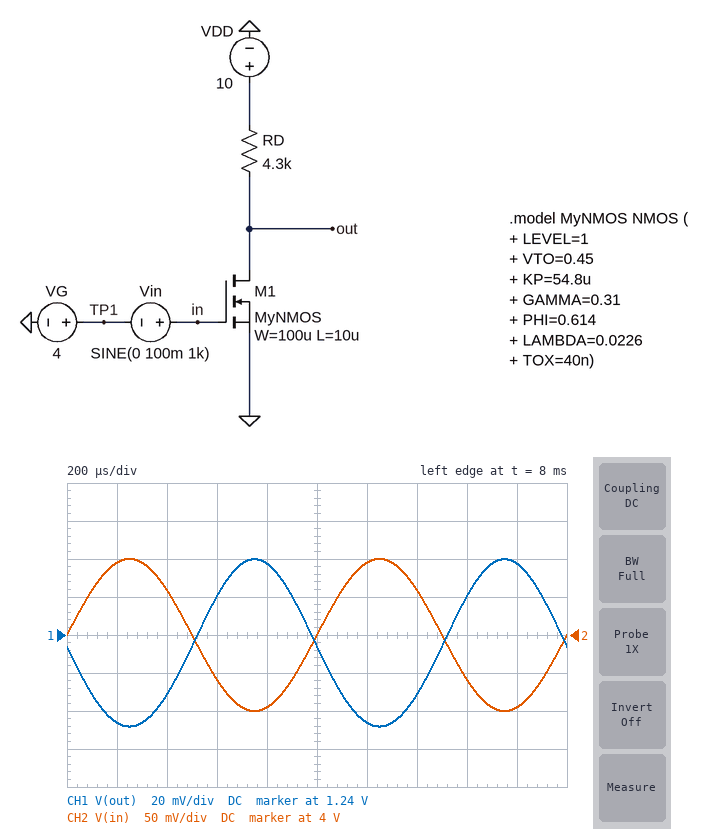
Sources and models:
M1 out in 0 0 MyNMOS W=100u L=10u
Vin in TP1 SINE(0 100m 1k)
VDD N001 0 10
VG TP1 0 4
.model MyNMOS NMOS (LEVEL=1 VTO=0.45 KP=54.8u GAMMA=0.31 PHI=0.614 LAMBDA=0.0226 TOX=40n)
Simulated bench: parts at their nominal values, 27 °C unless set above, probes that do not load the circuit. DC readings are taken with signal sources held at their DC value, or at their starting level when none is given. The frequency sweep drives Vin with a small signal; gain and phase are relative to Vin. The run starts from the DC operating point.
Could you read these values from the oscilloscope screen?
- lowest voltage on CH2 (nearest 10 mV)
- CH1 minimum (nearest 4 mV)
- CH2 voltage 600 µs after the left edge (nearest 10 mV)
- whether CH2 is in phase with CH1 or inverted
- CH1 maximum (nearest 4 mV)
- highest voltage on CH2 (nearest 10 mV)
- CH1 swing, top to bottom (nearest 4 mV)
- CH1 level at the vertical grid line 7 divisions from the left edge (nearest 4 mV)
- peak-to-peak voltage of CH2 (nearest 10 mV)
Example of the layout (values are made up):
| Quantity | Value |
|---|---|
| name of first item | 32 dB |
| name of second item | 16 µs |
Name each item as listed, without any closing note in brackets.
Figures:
| Quantity | Value |
|---|---|
| lowest voltage on CH2 | 3.90 V |
| CH1 minimum | 1.192 V |
| CH2 voltage 600 µs after the left edge | 3.94 V |
| whether CH2 is in phase with CH1 or inverted | inverted |
| CH1 maximum | 1.280 V |
| highest voltage on CH2 | 4.10 V |
| CH1 swing, top to bottom | 88 mV |
| CH1 level at the vertical grid line 7 divisions from the left edge | 1.208 V |
| peak-to-peak voltage of CH2 | 200 mV |
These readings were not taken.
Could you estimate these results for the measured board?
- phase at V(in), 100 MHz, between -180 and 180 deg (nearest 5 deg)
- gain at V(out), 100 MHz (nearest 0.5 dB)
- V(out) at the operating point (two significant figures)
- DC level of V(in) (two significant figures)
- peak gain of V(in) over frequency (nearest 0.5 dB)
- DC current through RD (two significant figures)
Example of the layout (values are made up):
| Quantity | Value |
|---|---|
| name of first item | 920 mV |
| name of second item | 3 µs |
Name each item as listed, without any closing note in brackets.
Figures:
| Quantity | Value |
|---|---|
| phase at V(in), 100 MHz, between -180 and 180 deg | 0 deg |
| gain at V(out), 100 MHz | -7.0 dB |
| V(out) at the operating point | 1.2 V |
| DC level of V(in) | 4.0 V |
| peak gain of V(in) over frequency | 0 dB |
| DC current through RD | 2.0 mA |
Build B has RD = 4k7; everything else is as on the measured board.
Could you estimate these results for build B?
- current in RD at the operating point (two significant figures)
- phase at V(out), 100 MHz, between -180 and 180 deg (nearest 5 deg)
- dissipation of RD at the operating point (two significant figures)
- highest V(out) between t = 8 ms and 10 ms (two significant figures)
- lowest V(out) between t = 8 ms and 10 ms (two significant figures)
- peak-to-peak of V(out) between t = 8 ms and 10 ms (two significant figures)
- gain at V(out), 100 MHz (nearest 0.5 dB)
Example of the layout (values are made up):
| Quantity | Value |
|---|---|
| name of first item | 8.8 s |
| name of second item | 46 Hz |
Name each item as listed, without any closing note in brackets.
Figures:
| Quantity | Value |
|---|---|
| current in RD at the operating point | 1.9 mA |
| phase at V(out), 100 MHz, between -180 and 180 deg | 150 deg |
| dissipation of RD at the operating point | 17 mW |
| highest V(out) between t = 8 ms and 10 ms | 1.2 V |
| lowest V(out) between t = 8 ms and 10 ms | 1.1 V |
| peak-to-peak of V(out) between t = 8 ms and 10 ms | 78 mV |
| gain at V(out), 100 MHz | -7.5 dB |
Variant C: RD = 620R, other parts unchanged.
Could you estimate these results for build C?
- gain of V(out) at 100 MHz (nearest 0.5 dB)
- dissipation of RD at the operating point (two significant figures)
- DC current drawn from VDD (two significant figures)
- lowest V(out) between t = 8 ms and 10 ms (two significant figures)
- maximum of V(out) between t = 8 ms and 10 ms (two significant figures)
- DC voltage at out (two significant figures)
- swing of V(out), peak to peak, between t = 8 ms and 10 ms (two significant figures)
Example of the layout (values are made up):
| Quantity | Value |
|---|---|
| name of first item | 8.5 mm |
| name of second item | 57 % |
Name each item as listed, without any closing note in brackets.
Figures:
| Quantity | Value |
|---|---|
| gain of V(out) at 100 MHz | 2.5 dB |
| dissipation of RD at the operating point | 10 mW |
| DC current drawn from VDD | 4.0 mA |
| lowest V(out) between t = 8 ms and 10 ms | 7.4 V |
| maximum of V(out) between t = 8 ms and 10 ms | 7.6 V |
| DC voltage at out | 7.5 V |
| swing of V(out), peak to peak, between t = 8 ms and 10 ms | 270 mV |
